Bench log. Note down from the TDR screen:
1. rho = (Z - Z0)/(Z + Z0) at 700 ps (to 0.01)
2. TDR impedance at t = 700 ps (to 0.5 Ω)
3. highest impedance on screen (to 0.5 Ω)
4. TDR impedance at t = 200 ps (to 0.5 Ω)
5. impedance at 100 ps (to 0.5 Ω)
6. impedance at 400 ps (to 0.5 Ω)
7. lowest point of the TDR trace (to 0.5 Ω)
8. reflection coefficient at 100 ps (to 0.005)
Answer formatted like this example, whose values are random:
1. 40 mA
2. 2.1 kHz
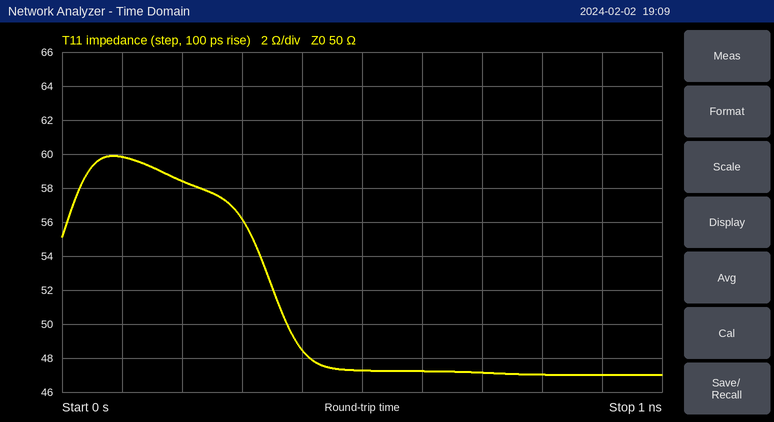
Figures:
1. -0.03
2. 47.0 Ω
3. 60.0 Ω
4. 58.5 Ω
5. 60.0 Ω
6. 48.5 Ω
7. 47.0 Ω
8. +0.090
